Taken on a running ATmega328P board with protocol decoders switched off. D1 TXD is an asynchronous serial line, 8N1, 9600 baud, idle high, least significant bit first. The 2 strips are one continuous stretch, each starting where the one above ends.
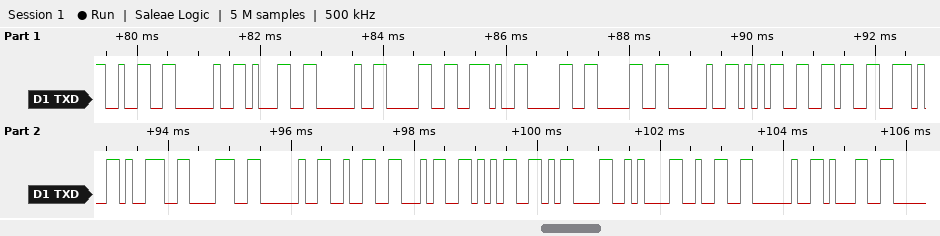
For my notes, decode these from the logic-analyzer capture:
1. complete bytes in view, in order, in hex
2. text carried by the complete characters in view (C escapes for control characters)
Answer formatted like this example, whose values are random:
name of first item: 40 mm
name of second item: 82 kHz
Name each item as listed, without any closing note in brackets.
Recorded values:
complete bytes in view, in order, in hex: 32 20 31 20 30 2E 30 30 20 35 36 2E 39 38 20 32 34 35 0D 0A 32 20 31
text carried by the complete characters in view: "2 1 0.00 56.98 245\r\n2 1"
